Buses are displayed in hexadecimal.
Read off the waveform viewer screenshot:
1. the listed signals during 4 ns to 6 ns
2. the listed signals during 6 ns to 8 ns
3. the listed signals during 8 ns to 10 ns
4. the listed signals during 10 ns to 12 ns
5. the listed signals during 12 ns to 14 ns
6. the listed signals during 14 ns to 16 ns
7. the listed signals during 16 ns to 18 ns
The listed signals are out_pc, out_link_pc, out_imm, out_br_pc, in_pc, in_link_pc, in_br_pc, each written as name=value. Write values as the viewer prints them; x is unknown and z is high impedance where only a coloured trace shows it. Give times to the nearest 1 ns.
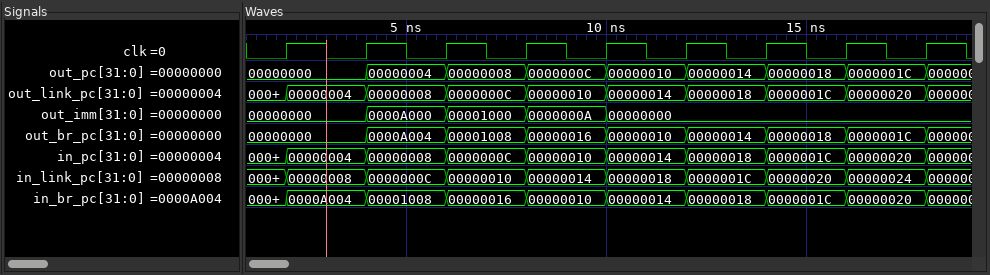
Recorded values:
out_pc=00000004, out_link_pc=00000008, out_imm=0000A000, out_br_pc=0000A004, in_pc=00000008, in_link_pc=0000000C, in_br_pc=00001008
out_pc=00000008, out_link_pc=0000000C, out_imm=00001000, out_br_pc=00001008, in_pc=0000000C, in_link_pc=00000010, in_br_pc=00000016
out_pc=0000000C, out_link_pc=00000010, out_imm=0000000A, out_br_pc=00000016, in_pc=00000010, in_link_pc=00000014, in_br_pc=00000010
out_pc=00000010, out_link_pc=00000014, out_imm=00000000, out_br_pc=00000010, in_pc=00000014, in_link_pc=00000018, in_br_pc=00000014
out_pc=00000014, out_link_pc=00000018, out_imm=00000000, out_br_pc=00000014, in_pc=00000018, in_link_pc=0000001C, in_br_pc=00000018
out_pc=00000018, out_link_pc=0000001C, out_imm=00000000, out_br_pc=00000018, in_pc=0000001C, in_link_pc=00000020, in_br_pc=0000001C
out_pc=0000001C, out_link_pc=00000020, out_imm=00000000, out_br_pc=0000001C, in_pc=00000020, in_link_pc=00000024, in_br_pc=00000020
